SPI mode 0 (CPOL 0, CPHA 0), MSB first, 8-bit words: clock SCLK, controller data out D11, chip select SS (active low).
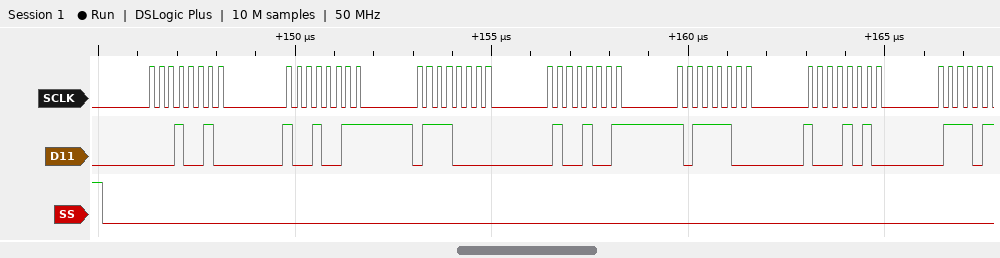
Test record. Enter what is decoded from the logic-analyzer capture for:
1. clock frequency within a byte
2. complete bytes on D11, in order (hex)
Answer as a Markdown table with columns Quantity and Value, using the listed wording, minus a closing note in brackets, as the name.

| Quantity | Value |
|---|---|
| clock frequency within a byte | 4 MHz |
| complete bytes on D11, in order | 12 93 70 49 BC 8A |
